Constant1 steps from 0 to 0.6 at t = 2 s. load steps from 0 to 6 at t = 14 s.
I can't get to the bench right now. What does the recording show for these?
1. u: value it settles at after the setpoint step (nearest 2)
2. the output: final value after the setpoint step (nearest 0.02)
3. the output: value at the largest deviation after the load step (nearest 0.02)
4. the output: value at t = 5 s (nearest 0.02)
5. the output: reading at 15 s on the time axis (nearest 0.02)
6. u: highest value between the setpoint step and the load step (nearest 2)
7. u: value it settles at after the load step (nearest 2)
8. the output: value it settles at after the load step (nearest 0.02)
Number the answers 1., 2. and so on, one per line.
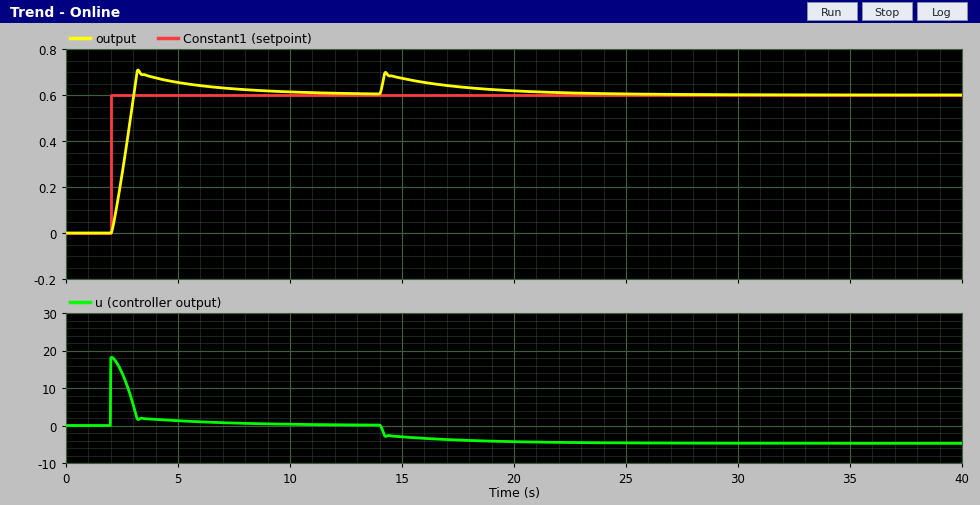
1. 0
2. 0.60
3. 0.70
4. 0.66
5. 0.68
6. 18
7. -4
8. 0.60
